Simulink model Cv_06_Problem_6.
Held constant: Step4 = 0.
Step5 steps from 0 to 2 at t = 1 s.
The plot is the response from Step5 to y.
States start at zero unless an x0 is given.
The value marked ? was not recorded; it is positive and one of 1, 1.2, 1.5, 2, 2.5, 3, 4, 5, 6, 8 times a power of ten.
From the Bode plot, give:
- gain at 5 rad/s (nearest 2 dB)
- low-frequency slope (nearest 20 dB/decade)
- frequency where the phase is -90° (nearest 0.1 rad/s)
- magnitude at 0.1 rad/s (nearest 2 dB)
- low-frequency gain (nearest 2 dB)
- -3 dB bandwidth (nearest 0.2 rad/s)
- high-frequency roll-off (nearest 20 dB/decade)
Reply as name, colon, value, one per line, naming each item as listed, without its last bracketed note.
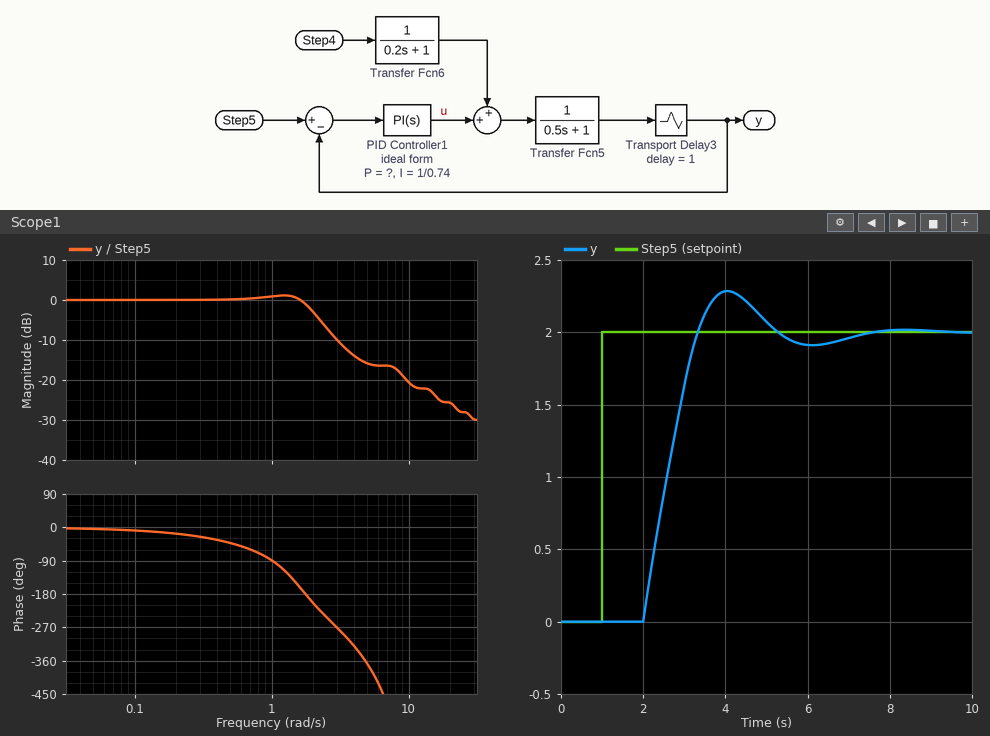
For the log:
gain at 5 rad/s: -16 dB
low-frequency slope: 0 dB/decade
frequency where the phase is -90°: 1.0 rad/s
magnitude at 0.1 rad/s: 0 dB
low-frequency gain: 0 dB
-3 dB bandwidth: 2.0 rad/s
high-frequency roll-off: -20 dB/decade
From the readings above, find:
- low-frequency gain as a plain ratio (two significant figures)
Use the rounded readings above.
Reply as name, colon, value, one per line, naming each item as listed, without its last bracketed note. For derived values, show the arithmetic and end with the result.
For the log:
low-frequency gain as a plain ratio: 10^(0 / 20) = 1.0
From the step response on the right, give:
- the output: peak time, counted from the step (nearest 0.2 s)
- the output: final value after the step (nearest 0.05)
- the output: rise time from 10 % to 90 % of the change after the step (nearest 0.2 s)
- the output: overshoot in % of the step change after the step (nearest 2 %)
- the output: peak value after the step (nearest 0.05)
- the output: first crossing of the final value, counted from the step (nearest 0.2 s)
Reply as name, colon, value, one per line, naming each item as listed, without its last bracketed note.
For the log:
the output: peak time, counted from the step: 3.0 s
the output: final value after the step: 2.00
the output: rise time from 10 % to 90 % of the change after the step: 1.0 s
the output: overshoot in % of the step change after the step: 14 %
the output: peak value after the step: 2.30
the output: first crossing of the final value, counted from the step: 2.4 s
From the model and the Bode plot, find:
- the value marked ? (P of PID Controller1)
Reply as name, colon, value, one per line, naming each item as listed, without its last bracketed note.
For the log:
the value marked ?: 0.5
